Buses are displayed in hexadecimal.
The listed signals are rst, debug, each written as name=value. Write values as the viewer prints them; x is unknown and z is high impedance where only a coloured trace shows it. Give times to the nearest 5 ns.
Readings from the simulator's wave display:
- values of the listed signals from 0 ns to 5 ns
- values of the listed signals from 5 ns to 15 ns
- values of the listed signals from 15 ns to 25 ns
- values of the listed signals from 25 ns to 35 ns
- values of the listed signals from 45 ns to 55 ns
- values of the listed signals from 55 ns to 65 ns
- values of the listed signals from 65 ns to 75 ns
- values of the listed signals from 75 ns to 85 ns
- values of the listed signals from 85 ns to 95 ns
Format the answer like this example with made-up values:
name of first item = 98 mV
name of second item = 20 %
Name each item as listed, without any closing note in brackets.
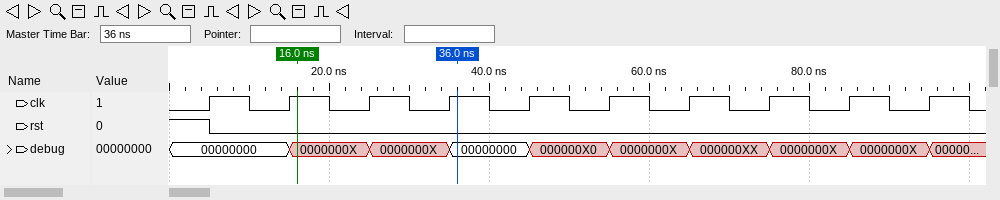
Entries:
values of the listed signals from 0 ns to 5 ns = rst=1, debug=00000000
values of the listed signals from 5 ns to 15 ns = rst=0, debug=00000000
values of the listed signals from 15 ns to 25 ns = rst=0, debug=0000000X
values of the listed signals from 25 ns to 35 ns = rst=0, debug=0000000X
values of the listed signals from 45 ns to 55 ns = rst=0, debug=000000X0
values of the listed signals from 55 ns to 65 ns = rst=0, debug=0000000X
values of the listed signals from 65 ns to 75 ns = rst=0, debug=000000XX
values of the listed signals from 75 ns to 85 ns = rst=0, debug=0000000X
values of the listed signals from 85 ns to 95 ns = rst=0, debug=0000000X
